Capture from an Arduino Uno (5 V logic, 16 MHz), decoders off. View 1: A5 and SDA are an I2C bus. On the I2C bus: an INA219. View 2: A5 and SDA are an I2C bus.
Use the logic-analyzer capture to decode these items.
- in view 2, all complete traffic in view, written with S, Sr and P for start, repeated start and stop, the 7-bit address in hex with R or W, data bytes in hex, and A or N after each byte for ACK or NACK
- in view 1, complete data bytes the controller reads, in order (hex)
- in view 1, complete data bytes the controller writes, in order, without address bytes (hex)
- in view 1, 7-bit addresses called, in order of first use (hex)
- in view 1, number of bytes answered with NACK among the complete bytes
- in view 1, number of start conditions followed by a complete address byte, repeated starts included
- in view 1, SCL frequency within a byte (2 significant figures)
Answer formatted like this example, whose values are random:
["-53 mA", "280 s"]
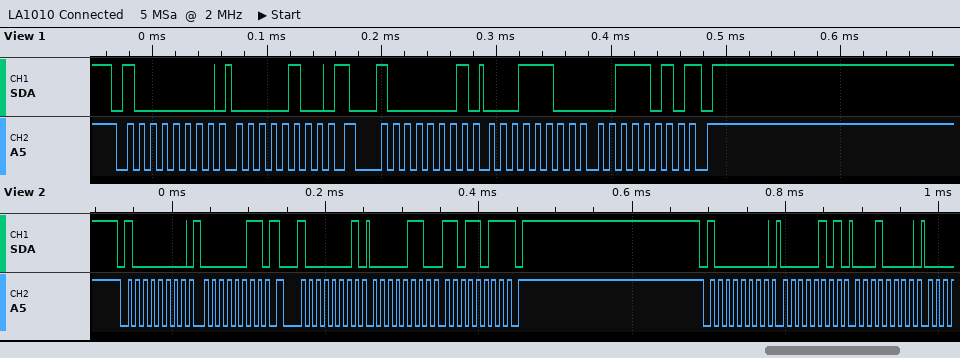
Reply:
["S 40W A 03 A Sr 40R A 06 A DB N P S 40W A 05 A 10 A", "1C 3A", "04", "0x40", "1", "2", "100 kHz"]
